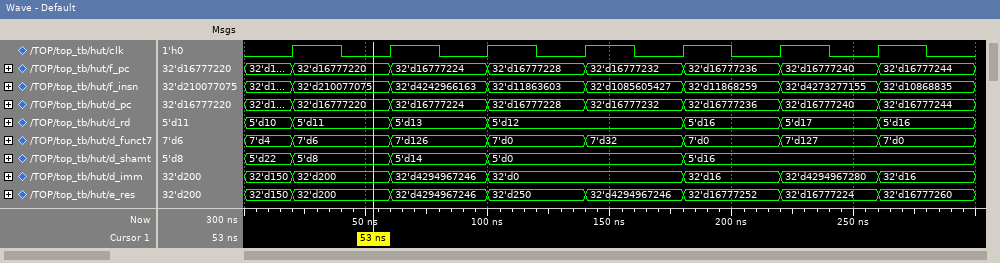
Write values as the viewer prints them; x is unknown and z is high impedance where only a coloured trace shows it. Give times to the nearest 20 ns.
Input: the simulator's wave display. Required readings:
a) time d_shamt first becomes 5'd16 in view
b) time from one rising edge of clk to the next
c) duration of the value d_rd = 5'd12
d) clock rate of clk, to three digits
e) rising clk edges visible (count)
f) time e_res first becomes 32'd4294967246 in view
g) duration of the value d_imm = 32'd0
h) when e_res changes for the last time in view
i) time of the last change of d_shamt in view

180 ns
40 ns
80 ns
25.0 MHz
7
60 ns
80 ns
260 ns
180 ns
